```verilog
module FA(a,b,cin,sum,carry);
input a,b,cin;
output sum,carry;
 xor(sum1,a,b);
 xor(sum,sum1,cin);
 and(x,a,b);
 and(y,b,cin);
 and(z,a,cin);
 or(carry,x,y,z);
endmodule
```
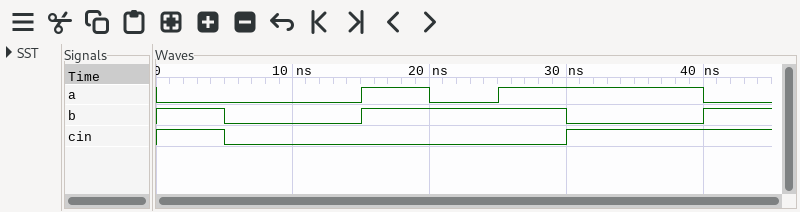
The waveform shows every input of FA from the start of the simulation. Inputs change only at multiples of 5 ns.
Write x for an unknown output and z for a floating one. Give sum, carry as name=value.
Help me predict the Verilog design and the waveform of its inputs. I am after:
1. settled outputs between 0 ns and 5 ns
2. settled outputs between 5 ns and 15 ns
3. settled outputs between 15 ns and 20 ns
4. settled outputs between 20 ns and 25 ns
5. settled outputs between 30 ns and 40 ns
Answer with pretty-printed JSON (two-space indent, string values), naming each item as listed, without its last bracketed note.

{
  "settled outputs between 0 ns and 5 ns": "sum=0, carry=1",
  "settled outputs between 5 ns and 15 ns": "sum=0, carry=0",
  "settled outputs between 15 ns and 20 ns": "sum=0, carry=1",
  "settled outputs between 20 ns and 25 ns": "sum=1, carry=0",
  "settled outputs between 30 ns and 40 ns": "sum=0, carry=1"
}
